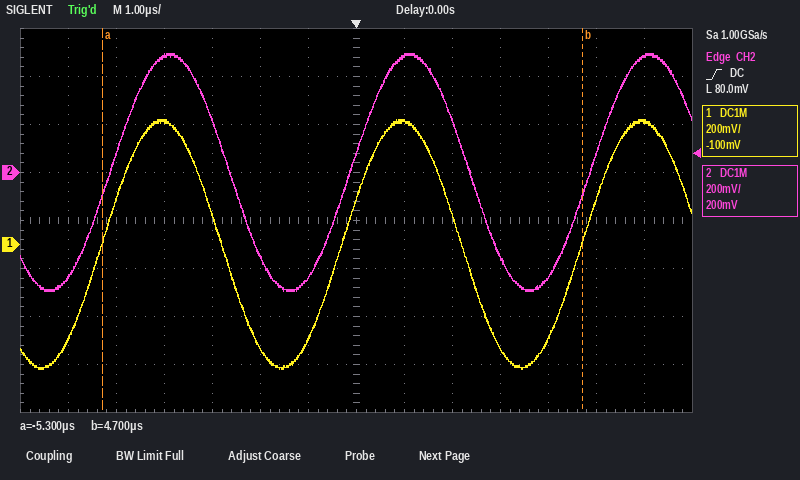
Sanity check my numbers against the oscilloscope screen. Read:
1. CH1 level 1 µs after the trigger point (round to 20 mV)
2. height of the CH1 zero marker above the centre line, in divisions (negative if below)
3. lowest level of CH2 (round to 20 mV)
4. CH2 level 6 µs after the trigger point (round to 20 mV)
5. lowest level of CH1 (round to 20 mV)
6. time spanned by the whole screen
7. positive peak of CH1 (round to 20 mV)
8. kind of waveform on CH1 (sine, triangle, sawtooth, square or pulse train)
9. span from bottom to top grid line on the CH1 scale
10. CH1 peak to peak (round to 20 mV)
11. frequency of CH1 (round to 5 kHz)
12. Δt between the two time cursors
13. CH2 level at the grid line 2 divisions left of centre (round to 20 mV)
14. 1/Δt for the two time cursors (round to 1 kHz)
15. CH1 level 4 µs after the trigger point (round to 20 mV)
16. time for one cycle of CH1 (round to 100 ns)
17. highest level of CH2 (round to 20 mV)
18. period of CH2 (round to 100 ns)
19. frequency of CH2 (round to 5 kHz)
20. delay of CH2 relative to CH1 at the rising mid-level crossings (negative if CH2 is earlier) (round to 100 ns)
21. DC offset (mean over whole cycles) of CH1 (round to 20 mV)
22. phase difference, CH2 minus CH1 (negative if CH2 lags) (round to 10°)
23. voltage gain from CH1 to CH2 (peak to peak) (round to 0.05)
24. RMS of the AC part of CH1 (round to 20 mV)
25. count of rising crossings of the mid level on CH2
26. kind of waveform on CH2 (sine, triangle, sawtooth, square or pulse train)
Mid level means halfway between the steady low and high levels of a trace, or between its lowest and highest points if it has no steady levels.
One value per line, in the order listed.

520 mV
-0.5 div
-500 mV
480 mV
-520 mV
14 µs
520 mV
sine
1.6 V
1.04 V
200 kHz
10.0 µs
-340 mV
100 kHz
-400 mV
5.0 µs
500 mV
5.0 µs
200 kHz
+200 ns
0 mV
-10°
0.95
360 mV
3
sine
